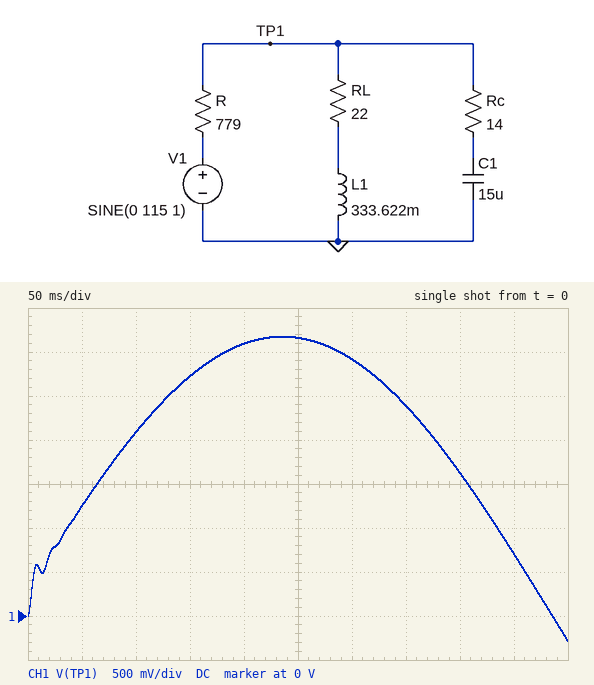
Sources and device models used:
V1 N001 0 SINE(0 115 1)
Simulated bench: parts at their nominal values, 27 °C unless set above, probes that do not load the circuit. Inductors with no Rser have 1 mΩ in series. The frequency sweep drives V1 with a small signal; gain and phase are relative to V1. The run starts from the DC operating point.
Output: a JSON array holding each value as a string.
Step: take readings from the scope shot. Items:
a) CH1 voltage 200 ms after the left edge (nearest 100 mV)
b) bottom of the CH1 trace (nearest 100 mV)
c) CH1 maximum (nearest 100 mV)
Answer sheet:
["3.1 V", "-300 mV", "3.2 V"]
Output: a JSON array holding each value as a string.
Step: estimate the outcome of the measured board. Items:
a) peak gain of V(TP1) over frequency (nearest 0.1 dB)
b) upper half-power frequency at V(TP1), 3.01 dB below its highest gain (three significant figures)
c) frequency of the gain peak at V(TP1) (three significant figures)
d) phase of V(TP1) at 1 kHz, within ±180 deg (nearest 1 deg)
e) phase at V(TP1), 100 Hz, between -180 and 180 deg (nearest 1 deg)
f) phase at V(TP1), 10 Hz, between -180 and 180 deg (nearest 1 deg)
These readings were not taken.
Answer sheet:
["-7.0 dB", "88.3 Hz", "71.5 Hz", "-36 deg", "-57 deg", "41 deg"]
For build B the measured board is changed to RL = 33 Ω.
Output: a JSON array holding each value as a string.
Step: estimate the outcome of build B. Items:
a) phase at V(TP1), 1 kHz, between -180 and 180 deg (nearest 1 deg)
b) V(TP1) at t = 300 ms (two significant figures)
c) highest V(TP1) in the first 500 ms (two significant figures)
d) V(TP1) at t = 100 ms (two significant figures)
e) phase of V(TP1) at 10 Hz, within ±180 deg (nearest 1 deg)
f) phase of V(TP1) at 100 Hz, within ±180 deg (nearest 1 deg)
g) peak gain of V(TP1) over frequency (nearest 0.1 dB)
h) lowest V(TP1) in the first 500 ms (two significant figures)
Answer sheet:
["-36 deg", "4.4 V", "4.7 V", "3.0 V", "29 deg", "-55 deg", "-8.3 dB", "-270 mV"]
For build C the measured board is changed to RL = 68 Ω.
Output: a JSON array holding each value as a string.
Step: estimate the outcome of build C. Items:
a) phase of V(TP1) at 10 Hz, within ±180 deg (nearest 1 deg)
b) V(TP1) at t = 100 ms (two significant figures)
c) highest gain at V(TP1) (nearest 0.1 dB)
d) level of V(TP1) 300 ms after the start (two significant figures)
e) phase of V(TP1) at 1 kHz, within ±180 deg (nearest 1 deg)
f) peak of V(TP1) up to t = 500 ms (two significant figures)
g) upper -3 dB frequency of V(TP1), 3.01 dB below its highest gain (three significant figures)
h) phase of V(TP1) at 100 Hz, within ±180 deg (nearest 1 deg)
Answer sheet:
["12 deg", "5.6 V", "-11.0 dB", "8.7 V", "-36 deg", "9.2 V", "102 Hz", "-52 deg"]
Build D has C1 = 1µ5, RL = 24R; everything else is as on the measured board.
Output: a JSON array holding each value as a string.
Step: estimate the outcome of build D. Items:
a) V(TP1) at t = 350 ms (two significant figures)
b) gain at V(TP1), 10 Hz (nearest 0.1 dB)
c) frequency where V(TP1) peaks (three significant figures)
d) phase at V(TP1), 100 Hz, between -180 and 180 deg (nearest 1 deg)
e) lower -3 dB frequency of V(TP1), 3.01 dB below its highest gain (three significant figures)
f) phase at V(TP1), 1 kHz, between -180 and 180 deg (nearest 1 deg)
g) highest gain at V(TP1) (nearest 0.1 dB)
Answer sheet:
["2.6 V", "-28.0 dB", "226 Hz", "64 deg", "163 Hz", "-74 deg", "-1.1 dB"]
